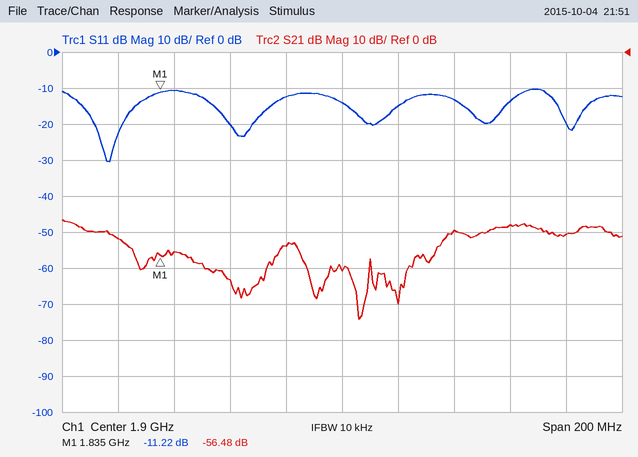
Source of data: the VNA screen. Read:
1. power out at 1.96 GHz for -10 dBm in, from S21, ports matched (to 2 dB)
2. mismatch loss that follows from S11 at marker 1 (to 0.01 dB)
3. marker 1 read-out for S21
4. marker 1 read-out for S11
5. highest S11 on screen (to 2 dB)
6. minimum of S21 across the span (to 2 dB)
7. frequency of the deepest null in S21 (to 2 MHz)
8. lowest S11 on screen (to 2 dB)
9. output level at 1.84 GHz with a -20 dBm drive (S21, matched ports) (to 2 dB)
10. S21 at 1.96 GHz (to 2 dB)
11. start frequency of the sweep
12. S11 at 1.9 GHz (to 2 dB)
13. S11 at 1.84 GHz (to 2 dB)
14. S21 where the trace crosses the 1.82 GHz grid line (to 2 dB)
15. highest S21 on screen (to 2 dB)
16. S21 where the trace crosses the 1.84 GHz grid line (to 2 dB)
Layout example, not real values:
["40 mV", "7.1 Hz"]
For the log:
["-58 dBm", "0.34 dB", "-56.48 dB", "-11.22 dB", "-10 dB", "-74 dB", "1.906 GHz", "-30 dB", "-76 dBm", "-48 dB", "1.8 GHz", "-14 dB", "-10 dB", "-52 dB", "-46 dB", "-56 dB"]
